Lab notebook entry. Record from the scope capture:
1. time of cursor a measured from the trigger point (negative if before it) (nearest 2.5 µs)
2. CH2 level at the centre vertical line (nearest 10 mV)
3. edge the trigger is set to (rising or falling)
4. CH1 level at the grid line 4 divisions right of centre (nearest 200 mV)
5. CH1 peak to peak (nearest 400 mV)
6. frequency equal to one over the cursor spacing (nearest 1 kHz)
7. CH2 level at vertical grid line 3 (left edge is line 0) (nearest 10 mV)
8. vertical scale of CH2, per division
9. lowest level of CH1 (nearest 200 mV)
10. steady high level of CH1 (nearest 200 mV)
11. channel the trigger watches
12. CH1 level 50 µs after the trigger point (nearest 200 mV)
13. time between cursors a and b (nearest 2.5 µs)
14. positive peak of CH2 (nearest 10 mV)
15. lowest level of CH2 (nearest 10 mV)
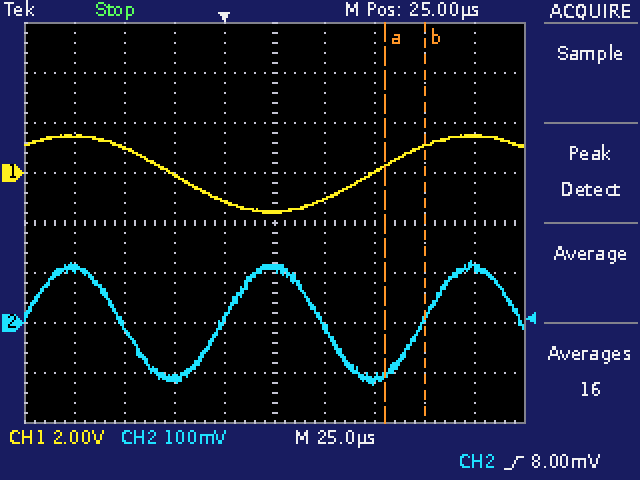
+80.0 µs
110 mV
rising
1.4 V
3.2 V
50 kHz
-110 mV
100 mV
-1.6 V
1.4 V
CH2
-1.0 V
20.0 µs
120 mV
-120 mV
